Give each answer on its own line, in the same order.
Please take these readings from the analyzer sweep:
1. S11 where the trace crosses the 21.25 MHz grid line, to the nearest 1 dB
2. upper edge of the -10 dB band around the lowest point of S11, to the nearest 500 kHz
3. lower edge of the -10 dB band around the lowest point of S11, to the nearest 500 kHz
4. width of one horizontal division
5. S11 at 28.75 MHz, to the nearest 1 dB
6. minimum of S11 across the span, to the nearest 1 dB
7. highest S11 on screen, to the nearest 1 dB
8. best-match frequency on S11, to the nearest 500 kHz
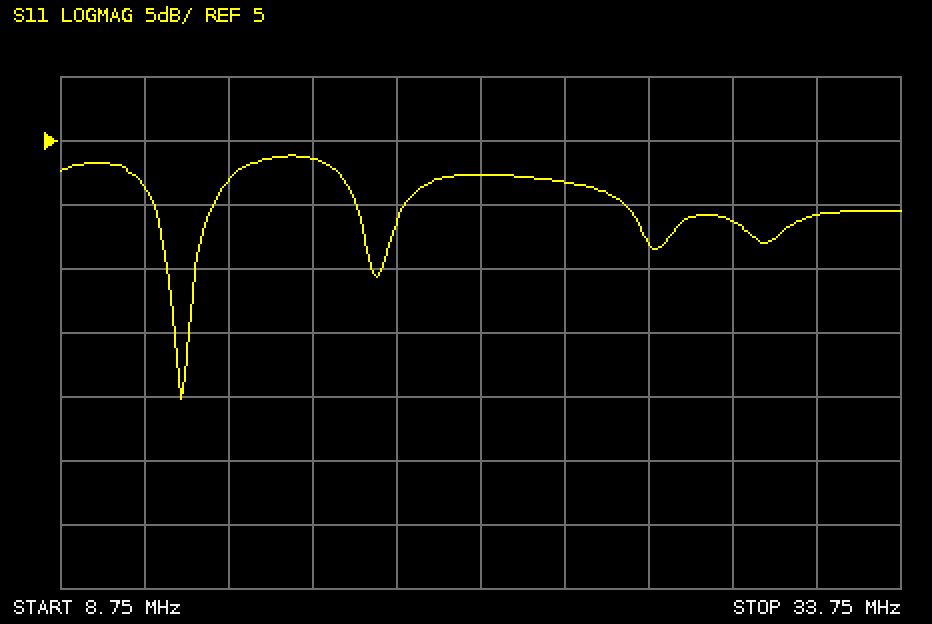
2 dB
12.5 MHz
12.0 MHz
2.5 MHz
-1 dB
-15 dB
4 dB
12.5 MHz
